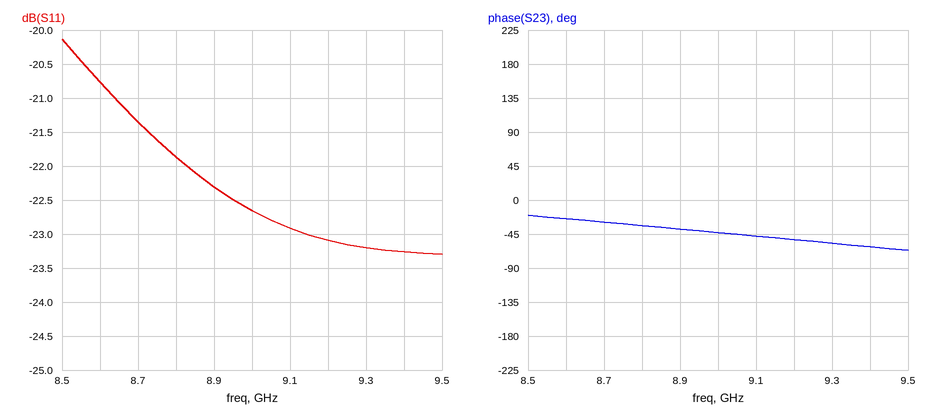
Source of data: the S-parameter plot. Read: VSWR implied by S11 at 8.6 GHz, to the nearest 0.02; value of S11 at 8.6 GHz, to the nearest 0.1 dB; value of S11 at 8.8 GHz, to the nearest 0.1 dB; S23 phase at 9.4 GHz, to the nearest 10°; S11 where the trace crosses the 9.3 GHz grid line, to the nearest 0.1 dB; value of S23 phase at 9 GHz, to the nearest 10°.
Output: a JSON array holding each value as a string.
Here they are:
["1.20", "-20.8 dB", "-21.9 dB", "-60°", "-23.2 dB", "-40°"]
